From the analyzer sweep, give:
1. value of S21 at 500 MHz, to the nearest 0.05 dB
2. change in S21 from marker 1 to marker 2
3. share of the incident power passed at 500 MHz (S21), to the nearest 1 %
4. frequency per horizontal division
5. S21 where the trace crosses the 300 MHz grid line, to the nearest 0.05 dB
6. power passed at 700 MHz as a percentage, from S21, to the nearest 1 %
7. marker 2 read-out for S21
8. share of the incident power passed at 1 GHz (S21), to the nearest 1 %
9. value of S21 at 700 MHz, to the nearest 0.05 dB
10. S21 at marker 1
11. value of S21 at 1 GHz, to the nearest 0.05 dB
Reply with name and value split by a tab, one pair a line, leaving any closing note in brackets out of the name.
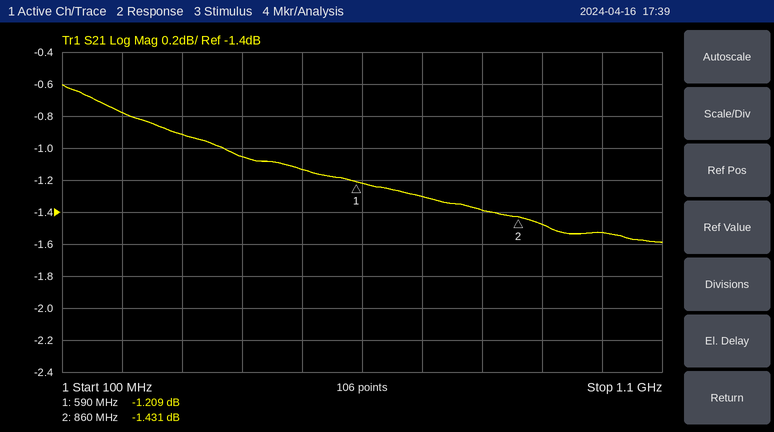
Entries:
value of S21 at 500 MHz, to the nearest 0.05 dB	-1.15 dB
change in S21 from marker 1 to marker 2	-0.222 dB
share of the incident power passed at 500 MHz (S21), to the nearest 1 %	77 %
frequency per horizontal division	100 MHz
S21 where the trace crosses the 300 MHz grid line, to the nearest 0.05 dB	-0.90 dB
power passed at 700 MHz as a percentage, from S21, to the nearest 1 %	74 %
marker 2 read-out for S21	-1.431 dB
share of the incident power passed at 1 GHz (S21), to the nearest 1 %	70 %
value of S21 at 700 MHz, to the nearest 0.05 dB	-1.30 dB
S21 at marker 1	-1.209 dB
value of S21 at 1 GHz, to the nearest 0.05 dB	-1.55 dB
